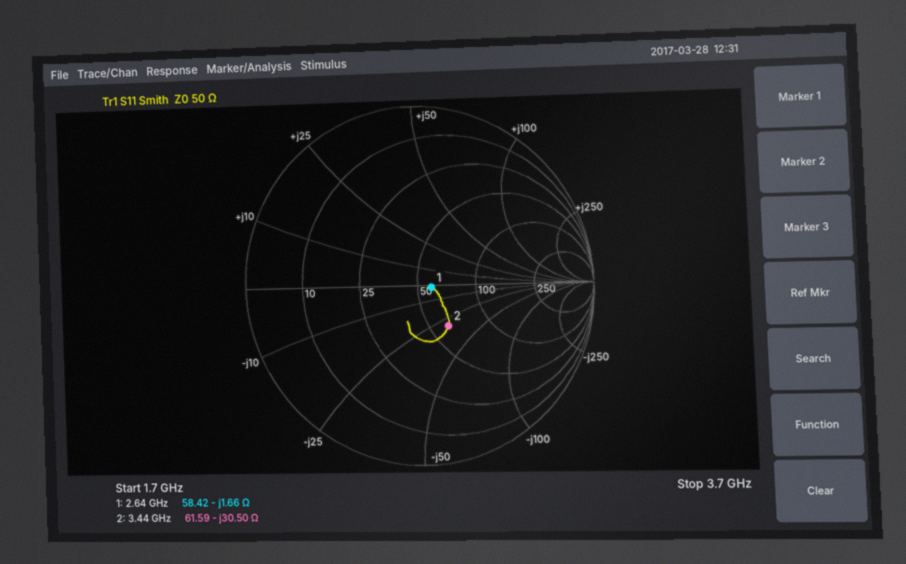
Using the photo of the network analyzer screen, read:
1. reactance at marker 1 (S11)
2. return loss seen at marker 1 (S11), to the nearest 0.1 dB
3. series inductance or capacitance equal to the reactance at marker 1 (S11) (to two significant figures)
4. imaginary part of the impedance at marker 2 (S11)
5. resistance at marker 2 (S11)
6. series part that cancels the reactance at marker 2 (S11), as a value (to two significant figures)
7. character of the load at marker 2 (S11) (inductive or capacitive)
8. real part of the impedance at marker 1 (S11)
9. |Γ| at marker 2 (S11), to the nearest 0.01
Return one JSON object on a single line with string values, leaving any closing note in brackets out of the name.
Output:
{"reactance at marker 1": "-1.66 Ω", "return loss seen at marker 1 (S11), to the nearest 0.1 dB": "22.0 dB", "series inductance or capacitance equal to the reactance at marker 1 (S11)": "36 pF", "imaginary part of the impedance at marker 2": "-30.50 Ω", "resistance at marker 2": "61.59 Ω", "series part that cancels the reactance at marker 2 (S11), as a value": "1.4 nH", "character of the load at marker 2 (S11)": "capacitive", "real part of the impedance at marker 1": "58.42 Ω", "|Γ| at marker 2 (S11), to the nearest 0.01": "0.28"}
